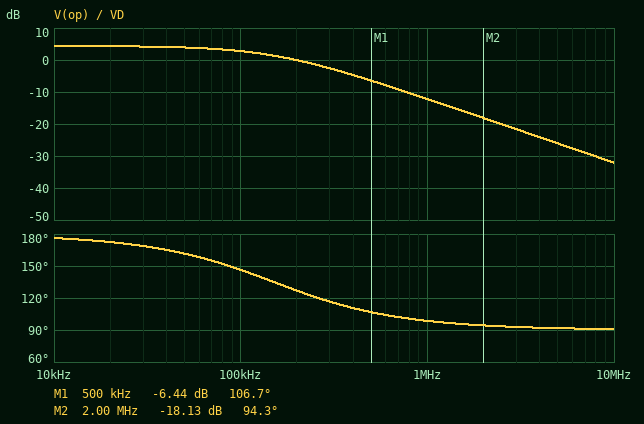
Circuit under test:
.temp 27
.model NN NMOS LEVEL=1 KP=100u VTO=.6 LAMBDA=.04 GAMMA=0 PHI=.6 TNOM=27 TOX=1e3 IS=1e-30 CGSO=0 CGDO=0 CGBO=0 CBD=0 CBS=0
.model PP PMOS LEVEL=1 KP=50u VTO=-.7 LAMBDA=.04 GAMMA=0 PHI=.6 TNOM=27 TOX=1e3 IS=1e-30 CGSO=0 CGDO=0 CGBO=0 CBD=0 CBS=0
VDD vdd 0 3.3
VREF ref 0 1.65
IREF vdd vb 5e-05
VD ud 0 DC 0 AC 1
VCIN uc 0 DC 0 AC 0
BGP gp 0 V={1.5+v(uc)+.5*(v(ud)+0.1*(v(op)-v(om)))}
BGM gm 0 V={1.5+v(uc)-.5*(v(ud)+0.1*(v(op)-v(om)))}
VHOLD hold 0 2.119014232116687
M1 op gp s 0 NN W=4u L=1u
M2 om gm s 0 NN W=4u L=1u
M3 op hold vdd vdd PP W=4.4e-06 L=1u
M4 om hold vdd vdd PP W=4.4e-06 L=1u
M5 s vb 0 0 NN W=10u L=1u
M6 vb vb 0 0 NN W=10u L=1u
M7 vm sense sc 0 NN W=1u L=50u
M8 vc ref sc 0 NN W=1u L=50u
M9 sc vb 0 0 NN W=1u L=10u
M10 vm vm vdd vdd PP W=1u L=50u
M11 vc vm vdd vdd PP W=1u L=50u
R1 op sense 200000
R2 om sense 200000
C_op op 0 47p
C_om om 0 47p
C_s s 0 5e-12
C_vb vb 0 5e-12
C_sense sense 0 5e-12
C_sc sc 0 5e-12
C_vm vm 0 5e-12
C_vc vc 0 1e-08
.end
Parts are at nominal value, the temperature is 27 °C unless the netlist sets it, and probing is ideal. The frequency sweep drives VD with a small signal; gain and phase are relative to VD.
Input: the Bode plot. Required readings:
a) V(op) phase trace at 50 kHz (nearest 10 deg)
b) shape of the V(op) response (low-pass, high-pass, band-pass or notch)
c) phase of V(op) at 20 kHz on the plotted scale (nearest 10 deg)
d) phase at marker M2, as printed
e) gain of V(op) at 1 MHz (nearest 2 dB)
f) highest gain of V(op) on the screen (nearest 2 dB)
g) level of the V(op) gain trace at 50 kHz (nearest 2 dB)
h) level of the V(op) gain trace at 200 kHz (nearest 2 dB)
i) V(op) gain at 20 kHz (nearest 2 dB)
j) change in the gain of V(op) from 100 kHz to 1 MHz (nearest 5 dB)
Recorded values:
160 deg
low-pass
170 deg
94.3 deg
-12 dB
4 dB
4 dB
0 dB
4 dB
-15 dB
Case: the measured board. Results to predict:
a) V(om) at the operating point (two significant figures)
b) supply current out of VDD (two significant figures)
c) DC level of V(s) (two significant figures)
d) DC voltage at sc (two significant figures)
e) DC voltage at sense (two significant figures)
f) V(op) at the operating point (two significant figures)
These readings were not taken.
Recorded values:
2.9 V
100 µA
560 mV
1.3 V
2.9 V
2.9 V
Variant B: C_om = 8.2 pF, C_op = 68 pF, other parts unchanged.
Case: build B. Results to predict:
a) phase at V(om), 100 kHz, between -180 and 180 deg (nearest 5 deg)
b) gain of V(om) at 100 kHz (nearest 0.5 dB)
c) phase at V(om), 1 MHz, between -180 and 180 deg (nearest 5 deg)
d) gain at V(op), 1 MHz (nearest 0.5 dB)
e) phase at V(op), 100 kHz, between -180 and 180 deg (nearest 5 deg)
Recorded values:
-5 deg
6.0 dB
-55 deg
-16.0 dB
130 deg
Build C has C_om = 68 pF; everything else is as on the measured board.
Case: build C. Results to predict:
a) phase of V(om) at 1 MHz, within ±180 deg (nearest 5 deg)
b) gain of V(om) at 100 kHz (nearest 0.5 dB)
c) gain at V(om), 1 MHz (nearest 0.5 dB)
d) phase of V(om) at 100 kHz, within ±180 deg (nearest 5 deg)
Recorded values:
-85 deg
1.0 dB
-15.5 dB
-45 deg
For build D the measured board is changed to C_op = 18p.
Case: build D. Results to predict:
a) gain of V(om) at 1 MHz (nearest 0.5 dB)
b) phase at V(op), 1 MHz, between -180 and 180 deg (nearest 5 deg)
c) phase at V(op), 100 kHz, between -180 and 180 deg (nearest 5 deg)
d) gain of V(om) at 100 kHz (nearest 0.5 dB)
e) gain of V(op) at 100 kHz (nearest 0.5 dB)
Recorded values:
-12.5 dB
110 deg
170 deg
2.0 dB
5.0 dB
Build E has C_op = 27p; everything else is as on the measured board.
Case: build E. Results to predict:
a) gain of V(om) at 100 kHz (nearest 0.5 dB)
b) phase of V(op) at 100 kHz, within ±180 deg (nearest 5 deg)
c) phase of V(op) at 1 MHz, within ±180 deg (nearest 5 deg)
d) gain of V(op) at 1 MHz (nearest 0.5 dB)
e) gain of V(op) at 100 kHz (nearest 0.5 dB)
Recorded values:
2.0 dB
160 deg
105 deg
-7.5 dB
4.5 dB
